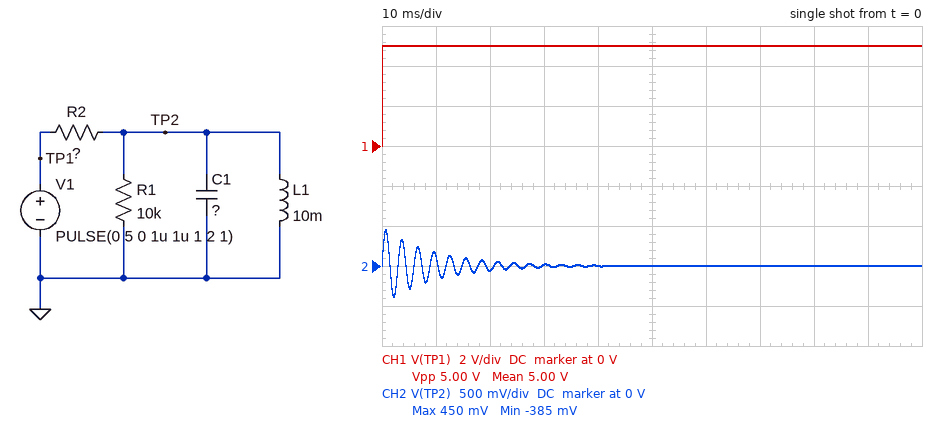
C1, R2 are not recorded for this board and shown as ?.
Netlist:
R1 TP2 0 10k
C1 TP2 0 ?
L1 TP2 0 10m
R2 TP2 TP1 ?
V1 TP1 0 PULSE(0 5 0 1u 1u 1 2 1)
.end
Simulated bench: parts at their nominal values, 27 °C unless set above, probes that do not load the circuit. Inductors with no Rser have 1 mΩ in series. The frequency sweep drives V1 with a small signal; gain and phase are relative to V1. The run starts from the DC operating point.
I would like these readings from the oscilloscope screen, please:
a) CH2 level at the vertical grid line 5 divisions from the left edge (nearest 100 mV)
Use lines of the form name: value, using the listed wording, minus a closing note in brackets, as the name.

CH2 level at the vertical grid line 5 divisions from the left edge: 0 V
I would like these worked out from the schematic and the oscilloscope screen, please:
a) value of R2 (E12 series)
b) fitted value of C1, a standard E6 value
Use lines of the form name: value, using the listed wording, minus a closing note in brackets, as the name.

value of R2: 220 Ω
fitted value of C1, a standard E6 value: 22 µF
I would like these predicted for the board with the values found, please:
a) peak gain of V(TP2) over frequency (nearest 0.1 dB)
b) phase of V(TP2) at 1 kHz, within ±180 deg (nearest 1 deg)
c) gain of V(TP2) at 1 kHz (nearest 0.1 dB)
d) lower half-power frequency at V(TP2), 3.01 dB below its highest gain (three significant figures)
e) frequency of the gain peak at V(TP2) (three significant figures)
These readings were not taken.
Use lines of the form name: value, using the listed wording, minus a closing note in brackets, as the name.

peak gain of V(TP2) over frequency: -0.2 dB
phase of V(TP2) at 1 kHz, within ±180 deg: -88 deg
gain of V(TP2) at 1 kHz: -28.6 dB
lower half-power frequency at V(TP2), 3.01 dB below its highest gain: 323 Hz
frequency of the gain peak at V(TP2): 339 Hz
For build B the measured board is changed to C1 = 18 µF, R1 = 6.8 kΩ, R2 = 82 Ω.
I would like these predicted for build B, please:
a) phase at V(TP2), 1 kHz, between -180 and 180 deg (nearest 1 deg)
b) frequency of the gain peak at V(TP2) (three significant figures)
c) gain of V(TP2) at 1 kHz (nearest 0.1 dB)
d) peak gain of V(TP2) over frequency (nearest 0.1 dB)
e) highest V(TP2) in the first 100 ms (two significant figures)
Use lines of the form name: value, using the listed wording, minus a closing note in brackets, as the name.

phase at V(TP2), 1 kHz, between -180 and 180 deg: -83 deg
frequency of the gain peak at V(TP2): 375 Hz
gain of V(TP2) at 1 kHz: -18.1 dB
peak gain of V(TP2) over frequency: -0.1 dB
highest V(TP2) in the first 100 ms: 1.2 V
